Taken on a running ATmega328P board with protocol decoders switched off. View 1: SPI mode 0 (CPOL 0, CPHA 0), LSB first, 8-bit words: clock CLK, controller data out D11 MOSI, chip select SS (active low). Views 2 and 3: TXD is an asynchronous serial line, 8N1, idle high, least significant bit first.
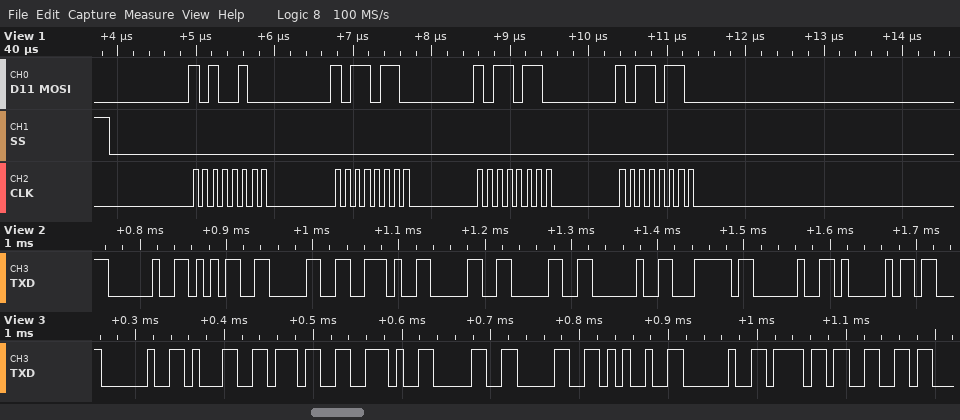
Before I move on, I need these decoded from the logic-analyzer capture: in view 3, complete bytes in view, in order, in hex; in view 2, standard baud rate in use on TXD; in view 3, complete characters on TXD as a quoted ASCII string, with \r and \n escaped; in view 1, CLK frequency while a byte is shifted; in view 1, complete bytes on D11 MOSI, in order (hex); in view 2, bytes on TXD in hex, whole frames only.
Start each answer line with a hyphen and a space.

- 20 31 37 2E 30 30 25 20 6F 66
- 115200 baud
- " 17.00% of"
- 8 MHz
- 25 6D 6D 6D
- 20 35 30 2E 30 30 20 7C 20 41
